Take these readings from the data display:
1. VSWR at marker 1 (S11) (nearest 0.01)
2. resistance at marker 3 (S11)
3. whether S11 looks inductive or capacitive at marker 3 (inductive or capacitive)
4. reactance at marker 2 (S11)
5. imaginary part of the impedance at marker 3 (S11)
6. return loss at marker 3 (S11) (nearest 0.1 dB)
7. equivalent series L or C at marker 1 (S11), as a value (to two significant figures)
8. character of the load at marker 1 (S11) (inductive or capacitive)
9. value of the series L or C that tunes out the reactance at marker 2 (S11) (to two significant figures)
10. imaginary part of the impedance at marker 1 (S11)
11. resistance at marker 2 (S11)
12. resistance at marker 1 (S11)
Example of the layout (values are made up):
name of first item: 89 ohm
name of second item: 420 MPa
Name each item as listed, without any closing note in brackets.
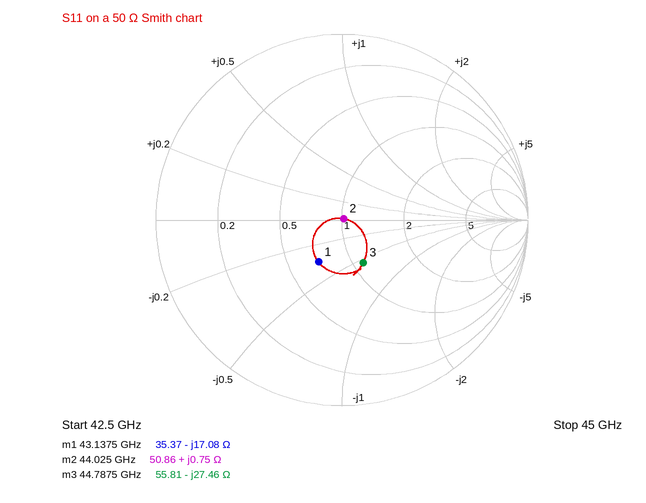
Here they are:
VSWR at marker 1 (S11): 1.70
resistance at marker 3: 55.81 Ω
whether S11 looks inductive or capacitive at marker 3: capacitive
reactance at marker 2: +0.75 Ω
imaginary part of the impedance at marker 3: -27.46 Ω
return loss at marker 3 (S11): 11.8 dB
equivalent series L or C at marker 1 (S11), as a value: 220 fF
character of the load at marker 1 (S11): capacitive
value of the series L or C that tunes out the reactance at marker 2 (S11): 4.8 pF
imaginary part of the impedance at marker 1: -17.08 Ω
resistance at marker 2: 50.86 Ω
resistance at marker 1: 35.37 Ω
